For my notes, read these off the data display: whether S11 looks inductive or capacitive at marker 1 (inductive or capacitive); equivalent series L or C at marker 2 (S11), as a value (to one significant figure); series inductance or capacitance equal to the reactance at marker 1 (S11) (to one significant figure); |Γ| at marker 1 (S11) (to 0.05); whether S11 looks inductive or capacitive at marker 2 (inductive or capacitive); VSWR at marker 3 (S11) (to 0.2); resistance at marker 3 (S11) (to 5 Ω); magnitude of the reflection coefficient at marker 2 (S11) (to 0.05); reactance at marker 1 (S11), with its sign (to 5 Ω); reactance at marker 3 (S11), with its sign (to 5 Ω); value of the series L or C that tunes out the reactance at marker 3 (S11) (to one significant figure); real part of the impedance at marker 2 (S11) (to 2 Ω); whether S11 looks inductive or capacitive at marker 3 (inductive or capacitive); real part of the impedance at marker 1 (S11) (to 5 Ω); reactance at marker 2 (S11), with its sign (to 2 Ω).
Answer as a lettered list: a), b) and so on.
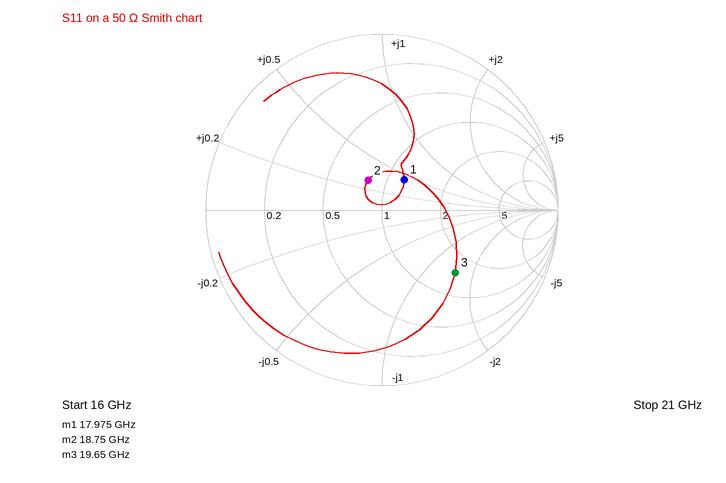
a) inductive
b) 100 pH
c) 200 pH
d) 0.20
e) inductive
f) 3.4
g) 75 Ω
h) 0.20
i) +20 Ω
j) -75 Ω
k) 600 pH
l) 40 Ω
m) capacitive
n) 60 Ω
o) +14 Ω
